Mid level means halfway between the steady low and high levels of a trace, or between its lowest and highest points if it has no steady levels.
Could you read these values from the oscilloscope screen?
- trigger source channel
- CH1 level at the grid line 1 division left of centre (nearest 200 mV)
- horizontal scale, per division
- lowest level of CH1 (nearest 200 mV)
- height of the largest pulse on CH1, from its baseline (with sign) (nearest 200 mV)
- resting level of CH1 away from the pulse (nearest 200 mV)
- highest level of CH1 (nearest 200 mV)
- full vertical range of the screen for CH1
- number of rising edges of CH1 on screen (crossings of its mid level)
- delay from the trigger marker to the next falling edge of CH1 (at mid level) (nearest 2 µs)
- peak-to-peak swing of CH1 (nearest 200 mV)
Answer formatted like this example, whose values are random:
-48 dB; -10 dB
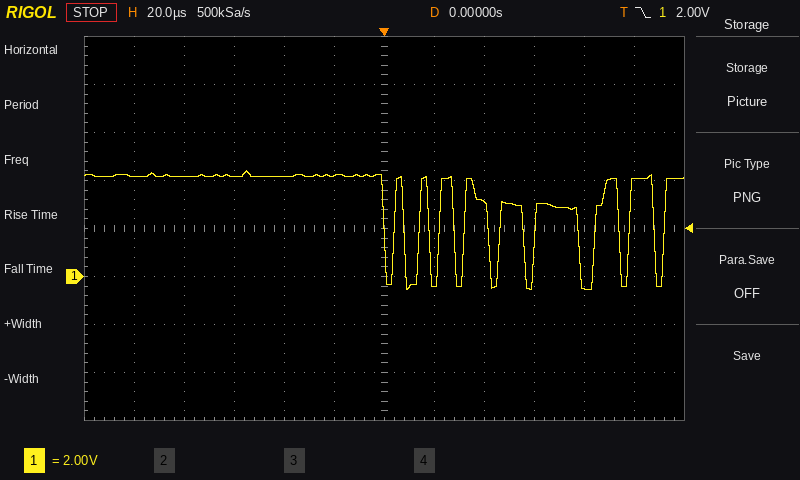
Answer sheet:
CH1; 4.2 V; 20 µs; -600 mV; -4.8 V; 4.2 V; 4.4 V; 16 V; 9; 8 µs; 5.0 V
